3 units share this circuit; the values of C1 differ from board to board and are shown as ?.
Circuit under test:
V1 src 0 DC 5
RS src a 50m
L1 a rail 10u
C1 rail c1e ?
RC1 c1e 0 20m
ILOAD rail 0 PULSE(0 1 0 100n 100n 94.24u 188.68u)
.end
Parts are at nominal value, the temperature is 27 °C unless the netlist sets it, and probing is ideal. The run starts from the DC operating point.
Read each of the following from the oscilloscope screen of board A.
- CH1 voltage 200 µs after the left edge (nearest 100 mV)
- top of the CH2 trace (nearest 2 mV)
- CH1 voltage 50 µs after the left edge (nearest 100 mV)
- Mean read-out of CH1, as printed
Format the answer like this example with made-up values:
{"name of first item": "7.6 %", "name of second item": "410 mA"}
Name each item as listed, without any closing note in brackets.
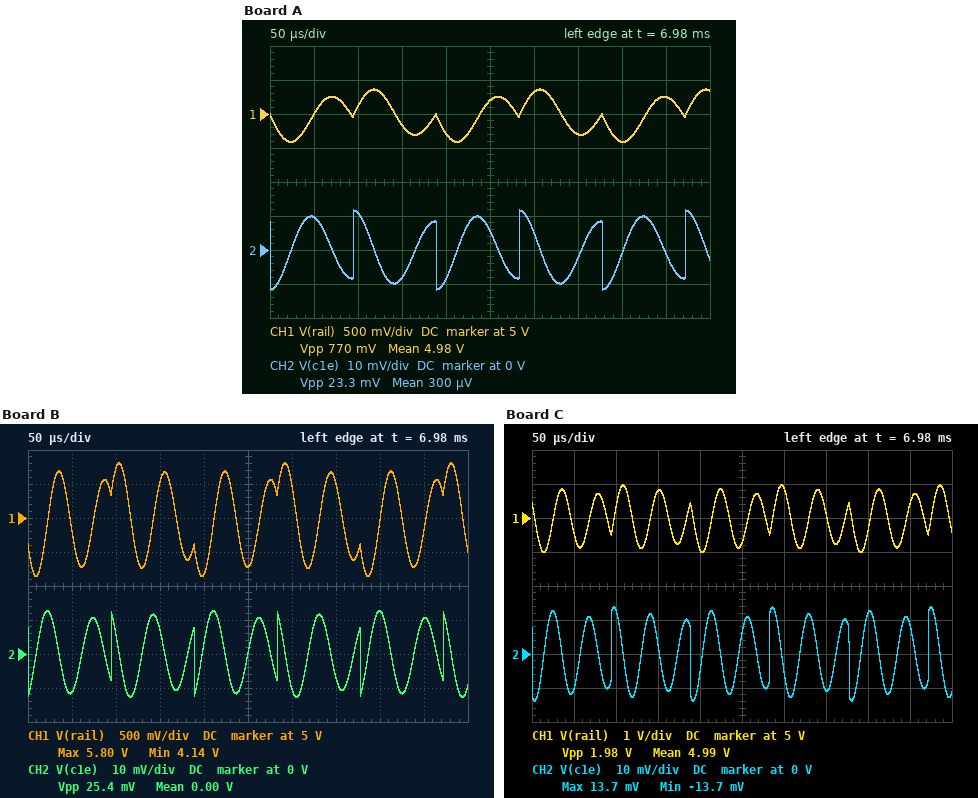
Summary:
{"CH1 voltage 200 µs after the left edge": "4.7 V", "top of the CH2 trace": "12 mV", "CH1 voltage 50 µs after the left edge": "5.0 V", "Mean read-out of CH1, as printed": "4.98 V"}
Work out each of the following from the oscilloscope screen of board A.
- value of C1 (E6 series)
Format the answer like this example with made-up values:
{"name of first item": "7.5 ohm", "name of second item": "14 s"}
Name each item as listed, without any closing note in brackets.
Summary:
{"value of C1": "22 µF"}
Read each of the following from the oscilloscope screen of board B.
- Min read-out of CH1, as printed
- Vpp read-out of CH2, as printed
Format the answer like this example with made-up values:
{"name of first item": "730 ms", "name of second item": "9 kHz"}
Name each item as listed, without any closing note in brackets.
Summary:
{"Min read-out of CH1, as printed": "4.14 V", "Vpp read-out of CH2, as printed": "25.4 mV"}
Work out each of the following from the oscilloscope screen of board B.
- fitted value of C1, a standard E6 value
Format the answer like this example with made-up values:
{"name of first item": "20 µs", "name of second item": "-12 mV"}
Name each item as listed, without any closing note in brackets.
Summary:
{"fitted value of C1, a standard E6 value": "6.8 µF"}
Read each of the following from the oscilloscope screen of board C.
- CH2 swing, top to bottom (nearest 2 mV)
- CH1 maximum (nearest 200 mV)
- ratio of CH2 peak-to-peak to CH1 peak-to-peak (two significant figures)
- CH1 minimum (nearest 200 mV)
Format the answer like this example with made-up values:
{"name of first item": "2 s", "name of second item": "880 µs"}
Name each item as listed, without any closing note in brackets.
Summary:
{"CH2 swing, top to bottom": "28 mV", "CH1 maximum": "6.0 V", "ratio of CH2 peak-to-peak to CH1 peak-to-peak": "0.014", "CH1 minimum": "4.0 V"}
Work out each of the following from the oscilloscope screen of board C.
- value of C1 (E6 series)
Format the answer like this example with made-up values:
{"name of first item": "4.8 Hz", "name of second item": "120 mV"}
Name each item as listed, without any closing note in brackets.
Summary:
{"value of C1": "4.7 µF"}
